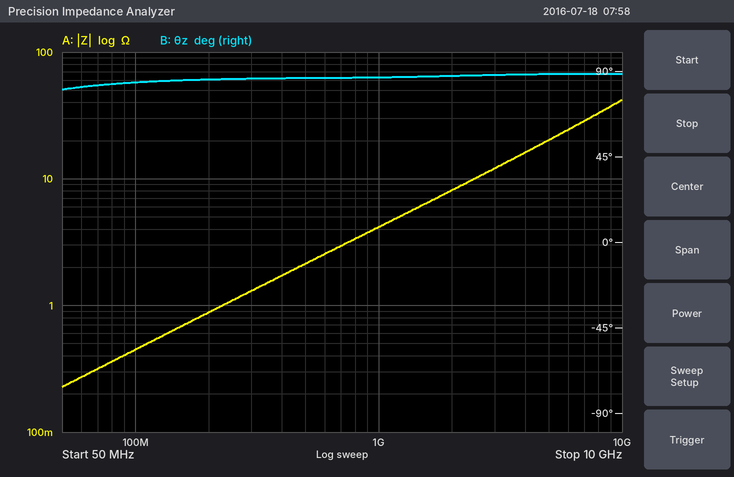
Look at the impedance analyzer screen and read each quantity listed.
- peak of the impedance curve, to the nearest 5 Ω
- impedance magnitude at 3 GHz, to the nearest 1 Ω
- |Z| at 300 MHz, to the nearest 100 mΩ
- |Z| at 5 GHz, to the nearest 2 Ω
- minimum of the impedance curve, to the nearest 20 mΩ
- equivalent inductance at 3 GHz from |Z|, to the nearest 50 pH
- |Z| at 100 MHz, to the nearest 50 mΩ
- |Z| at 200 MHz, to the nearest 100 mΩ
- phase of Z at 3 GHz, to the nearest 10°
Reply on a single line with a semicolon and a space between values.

40 Ω; 12 Ω; 1.3 Ω; 20 Ω; 220 mΩ; 650 pH; 450 mΩ; 900 mΩ; 90°
